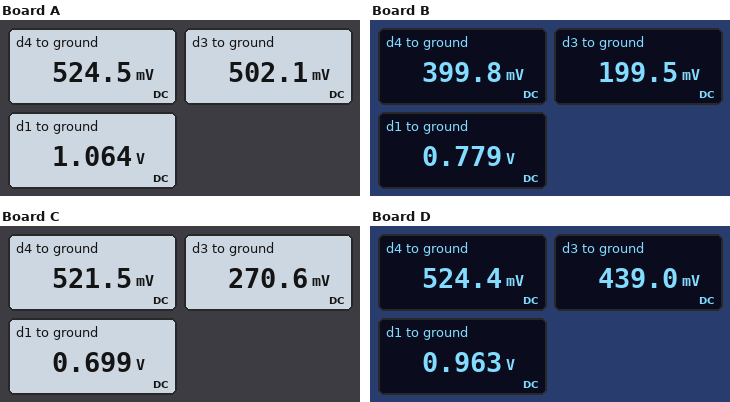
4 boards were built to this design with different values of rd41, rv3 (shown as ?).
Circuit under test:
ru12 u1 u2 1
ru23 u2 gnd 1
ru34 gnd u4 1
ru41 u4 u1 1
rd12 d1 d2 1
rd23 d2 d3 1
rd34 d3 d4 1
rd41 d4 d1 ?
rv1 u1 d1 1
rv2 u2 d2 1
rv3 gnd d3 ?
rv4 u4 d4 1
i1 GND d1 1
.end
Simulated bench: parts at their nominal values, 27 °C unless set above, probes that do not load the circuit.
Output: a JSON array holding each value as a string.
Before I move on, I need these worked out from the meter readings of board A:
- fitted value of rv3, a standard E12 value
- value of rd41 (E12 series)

["2.7 Ω", "3.3 Ω"]
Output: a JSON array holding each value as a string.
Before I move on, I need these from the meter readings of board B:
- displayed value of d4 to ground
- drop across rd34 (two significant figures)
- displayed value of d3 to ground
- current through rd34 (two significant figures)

["399.8 mV", "200 mV", "199.5 mV", "200 mA"]
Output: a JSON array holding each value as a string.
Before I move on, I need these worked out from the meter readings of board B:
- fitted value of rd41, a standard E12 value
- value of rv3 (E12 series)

["1.2 Ω", "0.47 Ω"]
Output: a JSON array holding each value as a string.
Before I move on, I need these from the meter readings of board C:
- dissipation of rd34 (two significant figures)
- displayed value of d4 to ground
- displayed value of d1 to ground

["63 mW", "521.5 mV", "0.699 V"]
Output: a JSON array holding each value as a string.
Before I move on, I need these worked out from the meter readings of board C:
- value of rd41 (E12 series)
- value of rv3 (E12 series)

["0.39 Ω", "0.68 Ω"]
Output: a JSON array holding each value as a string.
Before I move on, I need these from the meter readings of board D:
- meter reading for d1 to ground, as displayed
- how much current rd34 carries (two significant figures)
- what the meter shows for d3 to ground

["0.963 V", "85 mA", "439.0 mV"]
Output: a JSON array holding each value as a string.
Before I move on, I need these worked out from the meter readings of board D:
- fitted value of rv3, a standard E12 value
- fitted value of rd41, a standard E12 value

["1.8 Ω", "1.8 Ω"]
